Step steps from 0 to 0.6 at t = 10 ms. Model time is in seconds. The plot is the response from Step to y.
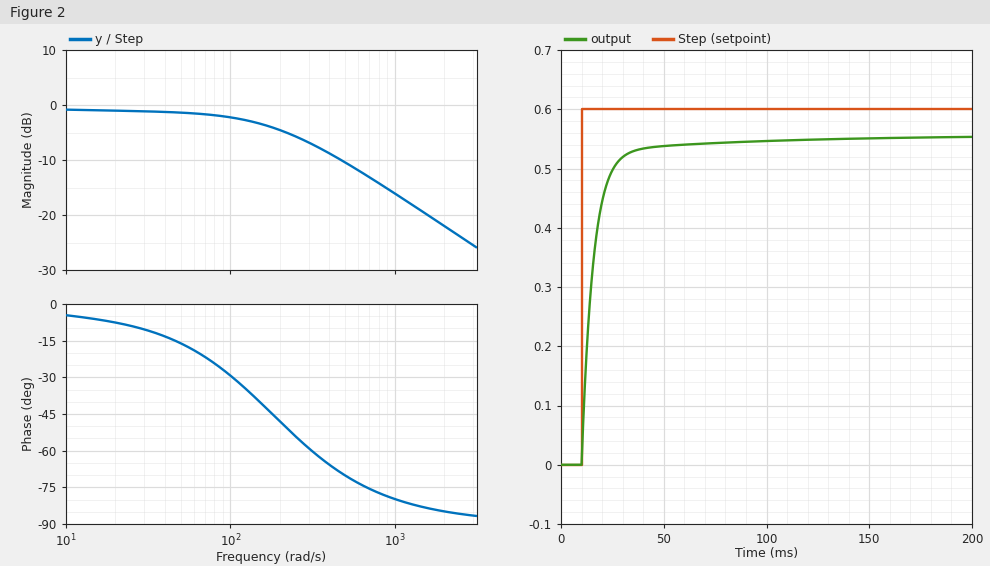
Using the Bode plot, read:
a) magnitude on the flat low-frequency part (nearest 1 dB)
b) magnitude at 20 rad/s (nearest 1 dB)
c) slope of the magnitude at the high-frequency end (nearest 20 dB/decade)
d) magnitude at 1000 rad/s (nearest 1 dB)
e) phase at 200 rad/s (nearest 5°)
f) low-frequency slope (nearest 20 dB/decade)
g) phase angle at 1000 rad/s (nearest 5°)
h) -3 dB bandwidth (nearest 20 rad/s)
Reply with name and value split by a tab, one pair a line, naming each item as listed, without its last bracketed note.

magnitude on the flat low-frequency part	-1 dB
magnitude at 20 rad/s	-1 dB
slope of the magnitude at the high-frequency end	-20 dB/decade
magnitude at 1000 rad/s	-16 dB
phase at 200 rad/s	-50°
low-frequency slope	0 dB/decade
phase angle at 1000 rad/s	-80°
-3 dB bandwidth	180 rad/s
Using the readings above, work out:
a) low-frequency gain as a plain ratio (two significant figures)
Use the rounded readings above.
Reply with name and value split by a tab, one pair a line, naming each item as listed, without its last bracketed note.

low-frequency gain as a plain ratio	0.89
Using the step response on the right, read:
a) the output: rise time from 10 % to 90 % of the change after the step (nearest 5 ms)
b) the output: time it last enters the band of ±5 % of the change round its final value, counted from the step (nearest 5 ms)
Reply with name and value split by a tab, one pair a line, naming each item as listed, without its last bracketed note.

the output: rise time from 10 % to 90 % of the change after the step	15 ms
the output: time it last enters the band of ±5 % of the change round its final value, counted from the step	25 ms
